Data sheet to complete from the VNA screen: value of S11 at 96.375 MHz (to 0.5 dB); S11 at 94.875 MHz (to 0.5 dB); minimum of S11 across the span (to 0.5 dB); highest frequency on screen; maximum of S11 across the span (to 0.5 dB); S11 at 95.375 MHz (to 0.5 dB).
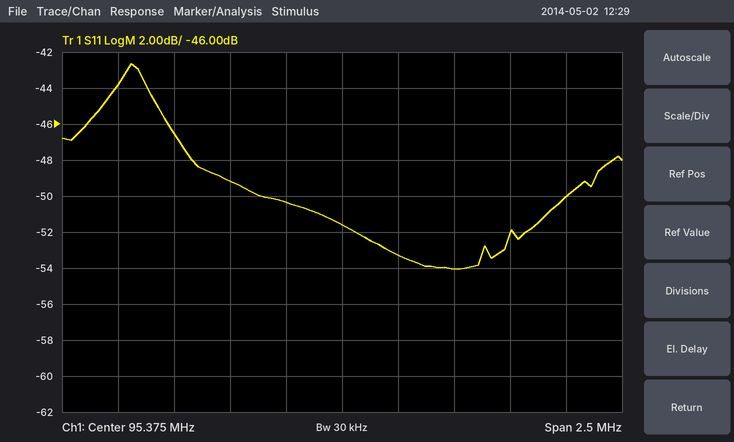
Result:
-50.0 dB
-49.0 dB
-54.0 dB
96.625 MHz
-42.5 dB
-51.5 dB
